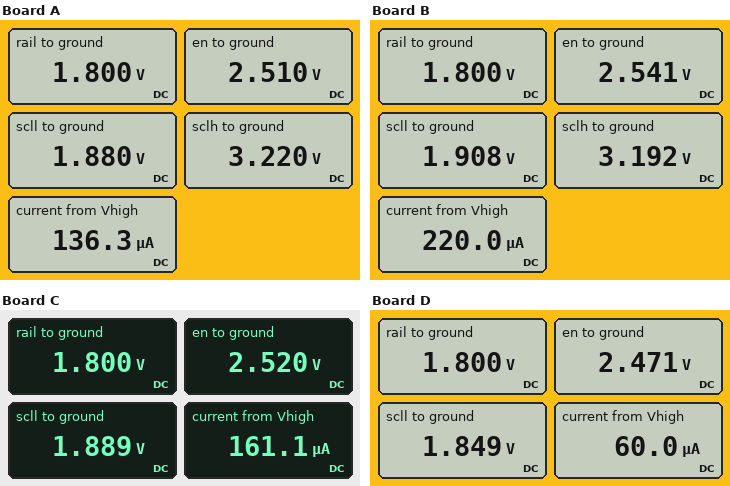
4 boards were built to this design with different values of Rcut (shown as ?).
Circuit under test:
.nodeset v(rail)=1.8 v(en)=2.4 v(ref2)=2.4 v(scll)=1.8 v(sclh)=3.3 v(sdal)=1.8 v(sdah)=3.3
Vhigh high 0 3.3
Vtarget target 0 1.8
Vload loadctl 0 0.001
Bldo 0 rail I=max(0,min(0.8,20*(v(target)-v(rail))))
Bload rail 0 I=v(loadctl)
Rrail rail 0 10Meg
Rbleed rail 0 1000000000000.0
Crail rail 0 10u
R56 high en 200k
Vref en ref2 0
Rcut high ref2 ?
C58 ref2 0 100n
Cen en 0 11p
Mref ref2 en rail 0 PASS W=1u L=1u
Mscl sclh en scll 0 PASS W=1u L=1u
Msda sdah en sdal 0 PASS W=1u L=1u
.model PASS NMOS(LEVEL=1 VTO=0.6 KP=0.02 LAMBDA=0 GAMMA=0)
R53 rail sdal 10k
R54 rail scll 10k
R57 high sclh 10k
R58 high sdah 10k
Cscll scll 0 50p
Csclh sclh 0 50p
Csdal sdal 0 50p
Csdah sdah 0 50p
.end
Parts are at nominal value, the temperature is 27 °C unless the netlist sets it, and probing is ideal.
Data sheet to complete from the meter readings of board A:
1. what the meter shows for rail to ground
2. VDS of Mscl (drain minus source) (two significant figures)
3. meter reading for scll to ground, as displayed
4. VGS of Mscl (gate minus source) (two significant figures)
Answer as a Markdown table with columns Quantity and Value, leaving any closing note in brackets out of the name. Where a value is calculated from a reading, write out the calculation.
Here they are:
| Quantity | Value |
|---|---|
| what the meter shows for rail to ground | 1.800 V |
| VDS of Mscl (drain minus source) | 3.22 V - 1.88 V = 1.3 V |
| meter reading for scll to ground, as displayed | 1.880 V |
| VGS of Mscl (gate minus source) | 2.51 V - 1.88 V = 630 mV |
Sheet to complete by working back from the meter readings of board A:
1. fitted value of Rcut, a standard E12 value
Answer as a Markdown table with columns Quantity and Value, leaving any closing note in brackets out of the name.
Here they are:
| Quantity | Value |
|---|---|
| fitted value of Rcut, a standard E12 value | 6.8 kΩ |
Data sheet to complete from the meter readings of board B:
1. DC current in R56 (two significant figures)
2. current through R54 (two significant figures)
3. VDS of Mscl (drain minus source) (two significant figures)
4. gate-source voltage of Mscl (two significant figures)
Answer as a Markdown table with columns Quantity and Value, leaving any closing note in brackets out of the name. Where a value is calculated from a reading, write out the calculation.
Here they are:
| Quantity | Value |
|---|---|
| DC current in R56 | (3.3 V - 2.541 V) / 200 kΩ = 3.8 µA |
| current through R54 | (1.908 V - 1.8 V) / 10 kΩ = 11 µA |
| VDS of Mscl (drain minus source) | 3.192 V - 1.908 V = 1.3 V |
| gate-source voltage of Mscl | 2.541 V - 1.908 V = 630 mV |
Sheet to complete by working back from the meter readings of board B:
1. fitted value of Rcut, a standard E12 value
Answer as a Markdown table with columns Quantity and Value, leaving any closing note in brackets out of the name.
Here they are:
| Quantity | Value |
|---|---|
| fitted value of Rcut, a standard E12 value | 3.9 kΩ |
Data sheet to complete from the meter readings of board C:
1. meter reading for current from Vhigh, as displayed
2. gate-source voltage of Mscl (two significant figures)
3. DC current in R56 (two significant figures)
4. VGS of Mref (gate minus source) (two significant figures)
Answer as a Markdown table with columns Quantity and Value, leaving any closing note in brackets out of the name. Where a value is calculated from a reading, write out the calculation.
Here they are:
| Quantity | Value |
|---|---|
| meter reading for current from Vhigh, as displayed | 161.1 µA |
| gate-source voltage of Mscl | 2.52 V - 1.889 V = 630 mV |
| DC current in R56 | (3.3 V - 2.52 V) / 200 kΩ = 3.9 µA |
| VGS of Mref (gate minus source) | 2.52 V - 1.8 V = 720 mV |
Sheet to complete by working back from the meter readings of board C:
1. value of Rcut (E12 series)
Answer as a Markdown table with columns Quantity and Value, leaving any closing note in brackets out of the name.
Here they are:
| Quantity | Value |
|---|---|
| value of Rcut | 5.6 kΩ |
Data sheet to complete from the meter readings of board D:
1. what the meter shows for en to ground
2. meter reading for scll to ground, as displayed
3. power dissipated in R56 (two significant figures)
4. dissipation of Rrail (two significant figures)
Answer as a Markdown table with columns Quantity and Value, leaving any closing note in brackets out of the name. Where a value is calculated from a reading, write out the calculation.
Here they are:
| Quantity | Value |
|---|---|
| what the meter shows for en to ground | 2.471 V |
| meter reading for scll to ground, as displayed | 1.849 V |
| power dissipated in R56 | (3.3 V - 2.471 V)^2 / 200 kΩ = 3.4 µW |
| dissipation of Rrail | (1.8 V)^2 / 10 MΩ = 320 nW |
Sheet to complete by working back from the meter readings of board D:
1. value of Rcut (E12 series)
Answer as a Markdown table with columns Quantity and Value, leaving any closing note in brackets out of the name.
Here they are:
| Quantity | Value |
|---|---|
| value of Rcut | 18 kΩ |
